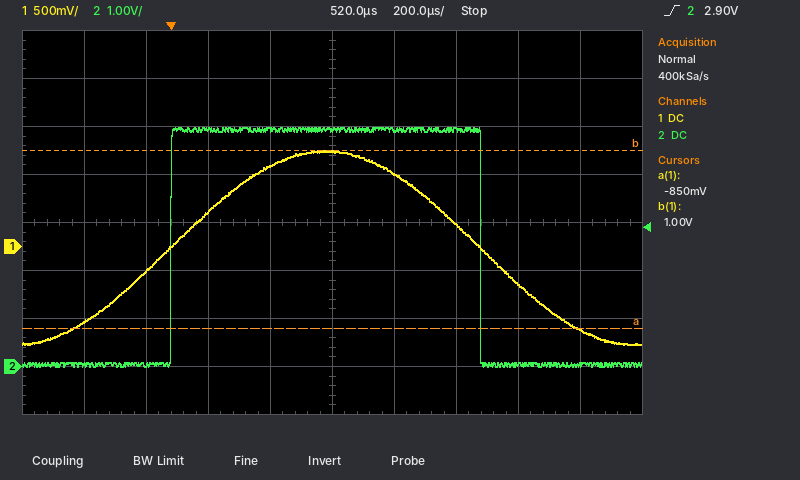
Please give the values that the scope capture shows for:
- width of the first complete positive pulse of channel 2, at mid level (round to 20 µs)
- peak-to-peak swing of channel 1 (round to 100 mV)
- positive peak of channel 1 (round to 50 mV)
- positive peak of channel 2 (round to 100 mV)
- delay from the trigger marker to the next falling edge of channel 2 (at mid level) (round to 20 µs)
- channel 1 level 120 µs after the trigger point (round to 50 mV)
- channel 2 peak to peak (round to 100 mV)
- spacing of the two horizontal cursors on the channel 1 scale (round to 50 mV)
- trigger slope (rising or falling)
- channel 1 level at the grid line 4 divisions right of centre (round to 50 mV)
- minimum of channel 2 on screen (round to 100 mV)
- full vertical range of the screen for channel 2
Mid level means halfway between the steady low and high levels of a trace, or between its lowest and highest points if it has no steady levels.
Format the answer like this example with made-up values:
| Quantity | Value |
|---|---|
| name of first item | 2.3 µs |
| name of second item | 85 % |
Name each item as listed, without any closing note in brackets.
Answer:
| Quantity | Value |
|---|---|
| width of the first complete positive pulse of channel 2, at mid level | 1.00 ms |
| peak-to-peak swing of channel 1 | 2.00 V |
| positive peak of channel 1 | 1.00 V |
| positive peak of channel 2 | 5.0 V |
| delay from the trigger marker to the next falling edge of channel 2 (at mid level) | 1.00 ms |
| channel 1 level 120 µs after the trigger point | 350 mV |
| channel 2 peak to peak | 5.0 V |
| spacing of the two horizontal cursors on the channel 1 scale | 1.85 V |
| trigger slope | rising |
| channel 1 level at the grid line 4 divisions right of centre | -850 mV |
| minimum of channel 2 on screen | 0.0 V |
| full vertical range of the screen for channel 2 | 8 V |
